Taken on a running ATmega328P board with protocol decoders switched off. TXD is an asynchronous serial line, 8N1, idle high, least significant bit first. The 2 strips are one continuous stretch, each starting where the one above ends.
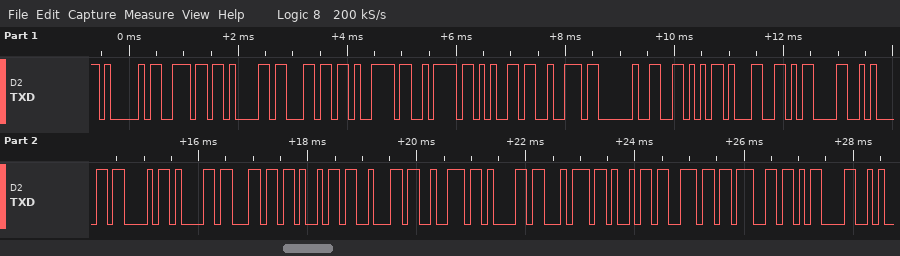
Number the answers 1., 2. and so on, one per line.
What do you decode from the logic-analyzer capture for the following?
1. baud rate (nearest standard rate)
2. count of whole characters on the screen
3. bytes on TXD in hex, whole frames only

1. 9600 baud
2. 25
3. 41 6E 61 6C 79 7A 65 72 20 56 31 0D 0A 43 61 6C 69 62 72 61 74 69 6E 67 0D
